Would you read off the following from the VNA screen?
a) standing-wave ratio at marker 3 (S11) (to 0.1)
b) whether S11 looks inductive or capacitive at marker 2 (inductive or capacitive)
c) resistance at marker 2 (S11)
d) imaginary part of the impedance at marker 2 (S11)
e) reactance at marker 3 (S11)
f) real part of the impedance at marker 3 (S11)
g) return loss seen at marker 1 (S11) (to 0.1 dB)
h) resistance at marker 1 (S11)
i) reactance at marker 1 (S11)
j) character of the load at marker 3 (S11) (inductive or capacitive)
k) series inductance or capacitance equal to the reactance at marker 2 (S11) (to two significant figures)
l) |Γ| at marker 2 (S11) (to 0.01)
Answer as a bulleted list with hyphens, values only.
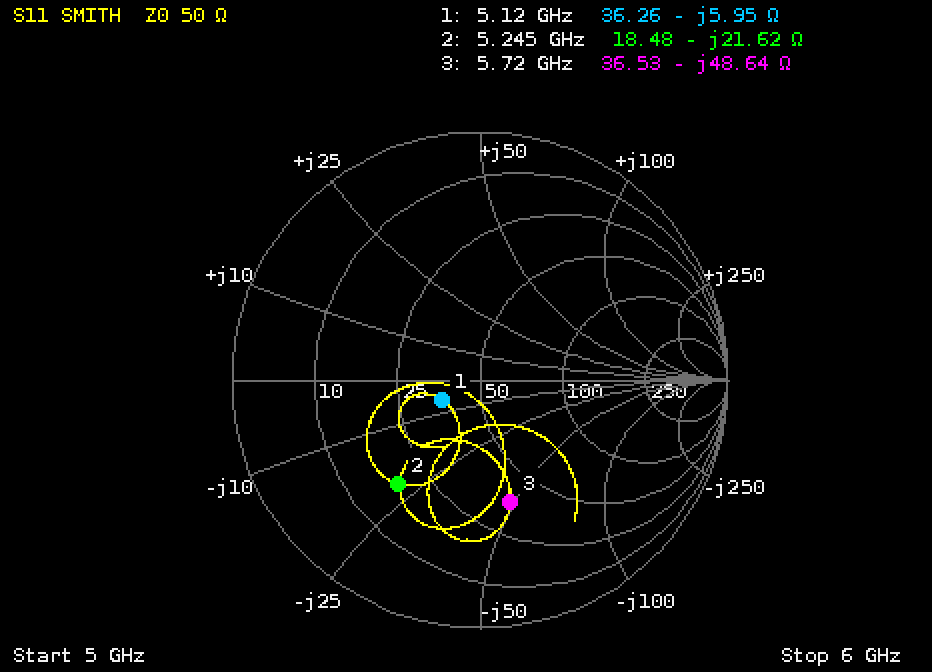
- 3.1
- capacitive
- 18.48 Ω
- -21.62 Ω
- -48.64 Ω
- 36.53 Ω
- 15.2 dB
- 36.26 Ω
- -5.95 Ω
- capacitive
- 1.4 pF
- 0.53
